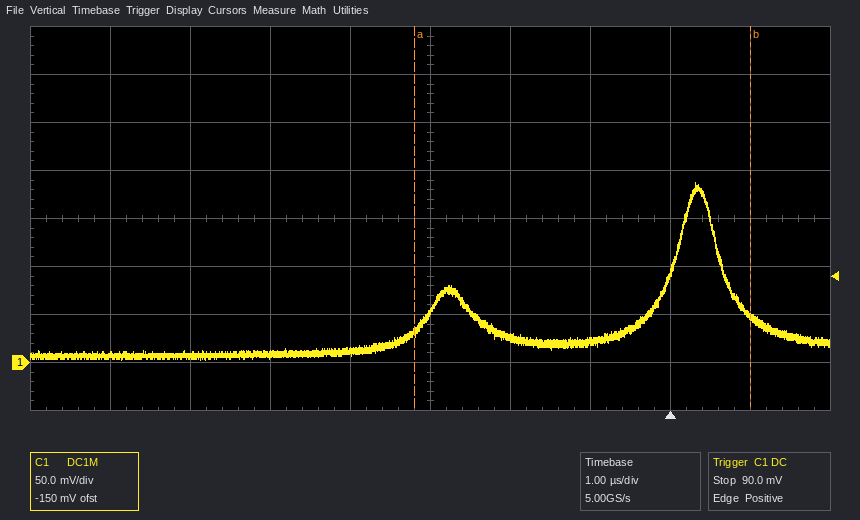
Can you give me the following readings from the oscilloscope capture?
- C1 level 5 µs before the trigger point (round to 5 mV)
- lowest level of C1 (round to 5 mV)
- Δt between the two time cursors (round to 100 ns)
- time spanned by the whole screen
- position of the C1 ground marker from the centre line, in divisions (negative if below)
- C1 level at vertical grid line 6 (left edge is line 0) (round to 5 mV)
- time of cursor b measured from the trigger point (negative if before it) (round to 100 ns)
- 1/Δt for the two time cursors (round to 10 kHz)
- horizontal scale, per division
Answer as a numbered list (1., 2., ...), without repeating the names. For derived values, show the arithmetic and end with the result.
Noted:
1. 10 mV
2. 0 mV
3. 4.2 µs
4. 10 µs
5. -3.0 div
6. 25 mV
7. +1.0 µs
8. 1 / 4.2 µs ≈ 240 kHz
9. 1 µs
